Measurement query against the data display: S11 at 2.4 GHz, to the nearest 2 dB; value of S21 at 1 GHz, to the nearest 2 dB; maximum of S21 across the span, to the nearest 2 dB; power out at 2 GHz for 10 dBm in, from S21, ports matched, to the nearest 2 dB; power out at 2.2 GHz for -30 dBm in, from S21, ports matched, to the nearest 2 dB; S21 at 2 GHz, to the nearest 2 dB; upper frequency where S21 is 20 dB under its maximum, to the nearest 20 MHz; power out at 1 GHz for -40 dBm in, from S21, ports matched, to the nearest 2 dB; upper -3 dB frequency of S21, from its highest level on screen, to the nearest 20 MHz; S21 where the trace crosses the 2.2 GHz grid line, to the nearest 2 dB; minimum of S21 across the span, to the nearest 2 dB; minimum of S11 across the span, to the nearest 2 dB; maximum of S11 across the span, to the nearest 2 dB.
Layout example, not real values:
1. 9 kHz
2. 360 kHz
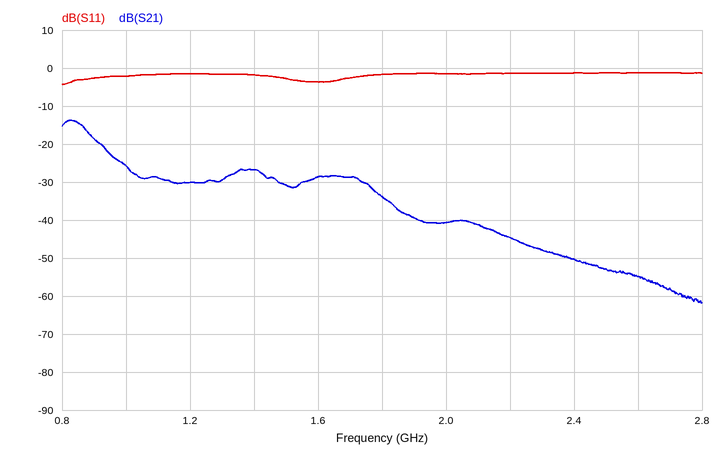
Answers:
1. -2 dB
2. -26 dB
3. -14 dB
4. -30 dBm
5. -74 dBm
6. -40 dB
7. 1.80 GHz
8. -66 dBm
9. 880 MHz
10. -44 dB
11. -62 dB
12. -4 dB
13. -2 dB
